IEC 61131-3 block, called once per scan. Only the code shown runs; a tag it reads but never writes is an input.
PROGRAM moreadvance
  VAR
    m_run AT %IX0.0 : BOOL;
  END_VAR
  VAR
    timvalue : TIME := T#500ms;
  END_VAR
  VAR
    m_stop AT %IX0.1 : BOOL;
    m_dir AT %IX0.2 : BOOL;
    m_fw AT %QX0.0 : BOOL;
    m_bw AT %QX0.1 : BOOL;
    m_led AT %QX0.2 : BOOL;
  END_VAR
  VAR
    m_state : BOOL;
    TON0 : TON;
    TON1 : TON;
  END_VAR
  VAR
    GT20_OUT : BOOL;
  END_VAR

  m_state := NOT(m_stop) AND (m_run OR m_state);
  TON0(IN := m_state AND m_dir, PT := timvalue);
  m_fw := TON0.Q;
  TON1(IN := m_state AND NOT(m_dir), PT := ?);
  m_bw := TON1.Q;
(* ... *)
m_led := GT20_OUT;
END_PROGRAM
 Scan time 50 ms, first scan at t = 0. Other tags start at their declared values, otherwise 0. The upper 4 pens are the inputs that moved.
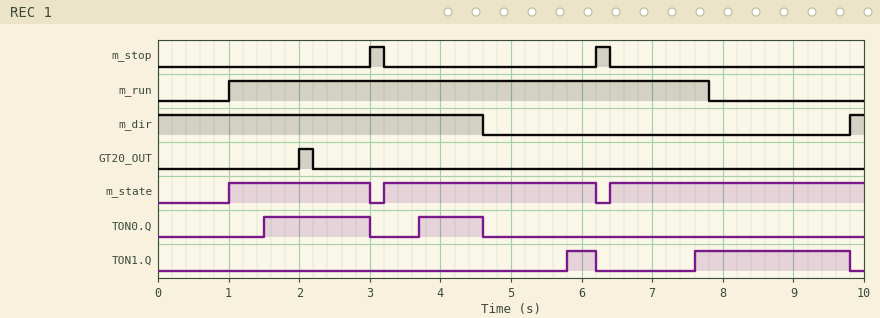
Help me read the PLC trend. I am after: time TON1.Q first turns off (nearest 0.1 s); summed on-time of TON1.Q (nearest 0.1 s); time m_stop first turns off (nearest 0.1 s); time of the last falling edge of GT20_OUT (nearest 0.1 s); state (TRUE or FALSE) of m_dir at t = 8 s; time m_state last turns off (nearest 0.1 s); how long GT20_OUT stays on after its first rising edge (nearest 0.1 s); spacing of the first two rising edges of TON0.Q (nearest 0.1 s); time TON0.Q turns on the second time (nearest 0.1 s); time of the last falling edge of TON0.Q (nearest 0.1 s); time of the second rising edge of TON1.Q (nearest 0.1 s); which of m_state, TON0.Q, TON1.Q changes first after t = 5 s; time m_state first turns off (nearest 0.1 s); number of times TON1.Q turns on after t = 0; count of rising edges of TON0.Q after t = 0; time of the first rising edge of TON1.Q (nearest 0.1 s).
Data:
6.2 s
2.6 s
3.2 s
2.2 s
FALSE
6.2 s
0.2 s
2.2 s
3.7 s
4.6 s
7.6 s
TON1.Q
3.0 s
2
2
5.8 s
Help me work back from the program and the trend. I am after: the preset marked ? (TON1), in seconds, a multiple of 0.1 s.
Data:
1.2 s
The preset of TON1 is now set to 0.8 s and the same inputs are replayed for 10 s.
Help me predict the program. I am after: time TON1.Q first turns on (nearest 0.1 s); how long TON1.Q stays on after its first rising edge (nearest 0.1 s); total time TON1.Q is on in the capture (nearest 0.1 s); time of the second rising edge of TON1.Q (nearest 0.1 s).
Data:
5.4 s
0.8 s
3.4 s
7.2 s
